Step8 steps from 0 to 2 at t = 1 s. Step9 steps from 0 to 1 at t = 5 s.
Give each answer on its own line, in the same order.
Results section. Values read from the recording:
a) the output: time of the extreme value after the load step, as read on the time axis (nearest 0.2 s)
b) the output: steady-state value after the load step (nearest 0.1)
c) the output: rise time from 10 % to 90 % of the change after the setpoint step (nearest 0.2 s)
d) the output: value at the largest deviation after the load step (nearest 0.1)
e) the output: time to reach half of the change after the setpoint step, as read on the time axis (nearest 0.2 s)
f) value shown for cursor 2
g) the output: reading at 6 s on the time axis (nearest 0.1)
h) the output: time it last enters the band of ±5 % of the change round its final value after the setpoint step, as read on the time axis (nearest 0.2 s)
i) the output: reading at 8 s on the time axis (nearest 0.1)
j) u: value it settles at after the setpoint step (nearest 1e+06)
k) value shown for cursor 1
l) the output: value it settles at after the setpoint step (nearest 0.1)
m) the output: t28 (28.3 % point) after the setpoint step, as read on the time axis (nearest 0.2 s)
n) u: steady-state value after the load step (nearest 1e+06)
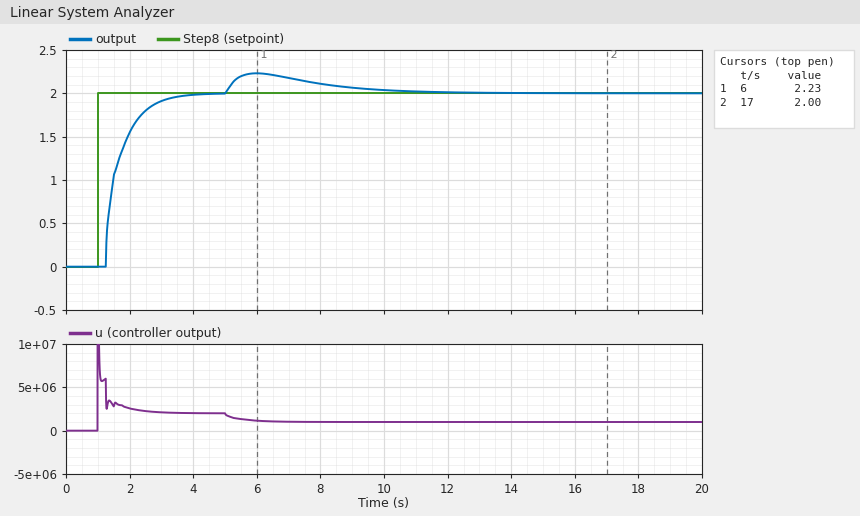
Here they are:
6.0 s
2.0
1.2 s
2.2
1.4 s
2.00
2.2
3.0 s
2.1
2000000
2.23
2.0
1.4 s
1000000
